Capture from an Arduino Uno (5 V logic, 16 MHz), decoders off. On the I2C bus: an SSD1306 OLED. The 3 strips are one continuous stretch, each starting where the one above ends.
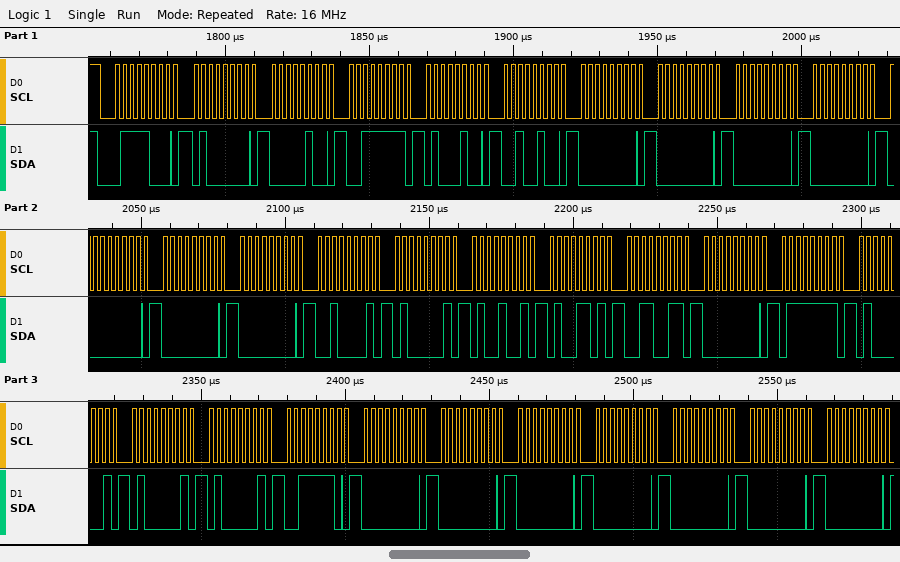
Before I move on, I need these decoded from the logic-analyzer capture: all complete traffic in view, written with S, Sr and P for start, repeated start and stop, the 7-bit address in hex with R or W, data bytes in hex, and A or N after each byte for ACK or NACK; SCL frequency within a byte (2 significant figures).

S 3CW A 40 A 04 A 3F A 44 A 24 A 00 A 00 A 00 A 00 A 00 A 00 A 00 A 21 A 41 A 49 A 4D A 33 A 00 A 7F A 41 A 41 A 41 A 3E A 00 A 00 A 00 A 00 A 00 A 00 A 00 A
400 kHz
